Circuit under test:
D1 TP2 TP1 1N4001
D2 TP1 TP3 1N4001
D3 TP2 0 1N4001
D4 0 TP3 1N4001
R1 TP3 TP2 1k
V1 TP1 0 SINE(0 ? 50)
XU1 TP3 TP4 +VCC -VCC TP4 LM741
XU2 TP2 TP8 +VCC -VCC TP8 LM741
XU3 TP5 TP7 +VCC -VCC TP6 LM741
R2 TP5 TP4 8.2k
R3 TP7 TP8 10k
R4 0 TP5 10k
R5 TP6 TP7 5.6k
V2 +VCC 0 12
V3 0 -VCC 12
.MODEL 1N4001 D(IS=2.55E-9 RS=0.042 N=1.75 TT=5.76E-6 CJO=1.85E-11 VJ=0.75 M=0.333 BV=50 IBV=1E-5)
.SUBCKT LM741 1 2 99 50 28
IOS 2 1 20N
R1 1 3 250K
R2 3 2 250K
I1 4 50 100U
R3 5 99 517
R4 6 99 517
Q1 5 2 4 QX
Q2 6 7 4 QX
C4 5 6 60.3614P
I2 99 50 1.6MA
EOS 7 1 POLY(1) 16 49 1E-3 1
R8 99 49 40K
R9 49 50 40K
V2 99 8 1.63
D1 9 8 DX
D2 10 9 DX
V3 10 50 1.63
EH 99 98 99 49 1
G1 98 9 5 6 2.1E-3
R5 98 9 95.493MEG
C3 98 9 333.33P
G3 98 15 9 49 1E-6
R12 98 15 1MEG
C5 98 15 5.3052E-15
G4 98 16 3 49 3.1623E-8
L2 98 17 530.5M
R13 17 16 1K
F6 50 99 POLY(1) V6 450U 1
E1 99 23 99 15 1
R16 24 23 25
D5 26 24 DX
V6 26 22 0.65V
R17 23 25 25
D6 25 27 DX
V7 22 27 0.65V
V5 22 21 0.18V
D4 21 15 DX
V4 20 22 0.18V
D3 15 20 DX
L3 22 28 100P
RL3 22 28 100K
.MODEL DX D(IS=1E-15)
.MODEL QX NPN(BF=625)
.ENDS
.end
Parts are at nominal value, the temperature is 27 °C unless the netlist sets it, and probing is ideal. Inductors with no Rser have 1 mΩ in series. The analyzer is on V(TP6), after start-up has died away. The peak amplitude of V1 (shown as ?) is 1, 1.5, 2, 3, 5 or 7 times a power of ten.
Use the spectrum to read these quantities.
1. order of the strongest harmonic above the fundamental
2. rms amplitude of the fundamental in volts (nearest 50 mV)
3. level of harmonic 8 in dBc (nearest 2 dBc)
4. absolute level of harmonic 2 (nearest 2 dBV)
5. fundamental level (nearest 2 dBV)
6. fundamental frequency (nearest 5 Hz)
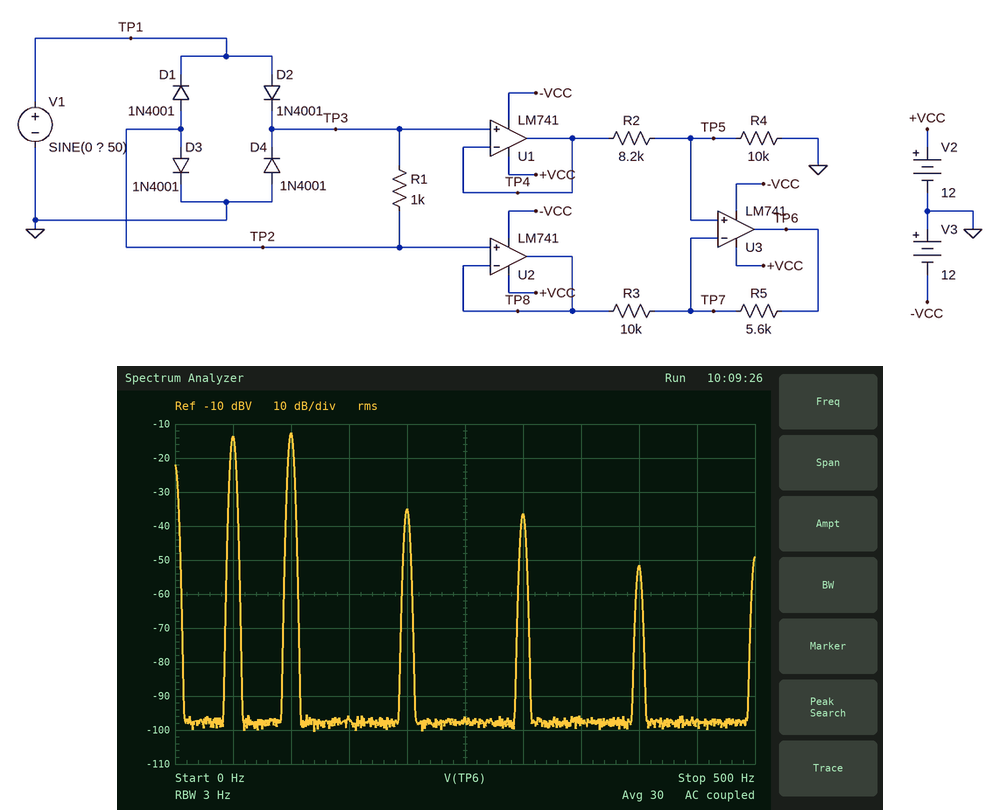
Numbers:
2
200 mV
-38 dBc
-12 dBV
-14 dBV
50 Hz
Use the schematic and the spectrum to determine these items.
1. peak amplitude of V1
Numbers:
2 V
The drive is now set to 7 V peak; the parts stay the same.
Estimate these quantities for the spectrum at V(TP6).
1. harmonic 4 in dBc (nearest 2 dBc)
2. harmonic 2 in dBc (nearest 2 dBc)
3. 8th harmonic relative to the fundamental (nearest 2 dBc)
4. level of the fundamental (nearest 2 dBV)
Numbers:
-10 dBc
6 dBc
-32 dBc
-2 dBV
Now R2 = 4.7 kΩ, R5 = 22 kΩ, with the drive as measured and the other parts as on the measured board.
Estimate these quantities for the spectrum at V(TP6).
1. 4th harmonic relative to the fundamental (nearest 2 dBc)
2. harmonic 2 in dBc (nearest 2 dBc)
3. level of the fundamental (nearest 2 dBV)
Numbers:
12 dBc
32 dBc
-36 dBV
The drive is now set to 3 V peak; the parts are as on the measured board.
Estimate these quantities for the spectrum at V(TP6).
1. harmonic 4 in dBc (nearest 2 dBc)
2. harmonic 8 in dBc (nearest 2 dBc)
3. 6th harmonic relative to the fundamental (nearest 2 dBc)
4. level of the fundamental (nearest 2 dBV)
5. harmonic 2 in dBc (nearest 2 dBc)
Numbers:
-22 dBc
-26 dBc
-26 dBc
-10 dBV
4 dBc
